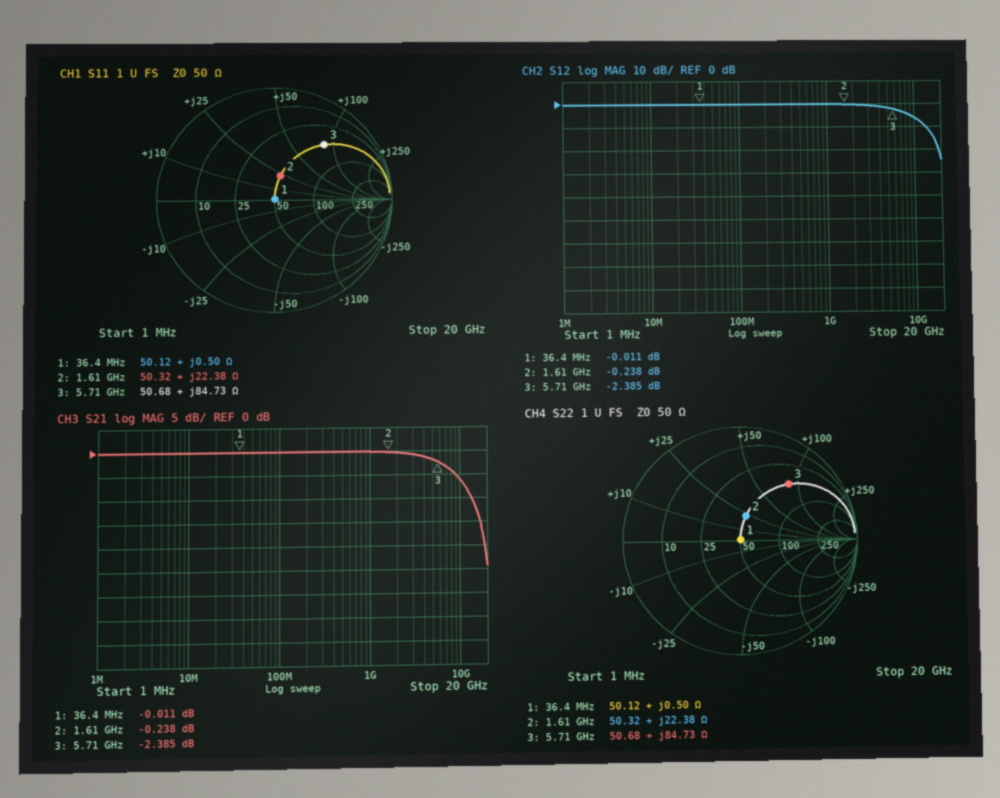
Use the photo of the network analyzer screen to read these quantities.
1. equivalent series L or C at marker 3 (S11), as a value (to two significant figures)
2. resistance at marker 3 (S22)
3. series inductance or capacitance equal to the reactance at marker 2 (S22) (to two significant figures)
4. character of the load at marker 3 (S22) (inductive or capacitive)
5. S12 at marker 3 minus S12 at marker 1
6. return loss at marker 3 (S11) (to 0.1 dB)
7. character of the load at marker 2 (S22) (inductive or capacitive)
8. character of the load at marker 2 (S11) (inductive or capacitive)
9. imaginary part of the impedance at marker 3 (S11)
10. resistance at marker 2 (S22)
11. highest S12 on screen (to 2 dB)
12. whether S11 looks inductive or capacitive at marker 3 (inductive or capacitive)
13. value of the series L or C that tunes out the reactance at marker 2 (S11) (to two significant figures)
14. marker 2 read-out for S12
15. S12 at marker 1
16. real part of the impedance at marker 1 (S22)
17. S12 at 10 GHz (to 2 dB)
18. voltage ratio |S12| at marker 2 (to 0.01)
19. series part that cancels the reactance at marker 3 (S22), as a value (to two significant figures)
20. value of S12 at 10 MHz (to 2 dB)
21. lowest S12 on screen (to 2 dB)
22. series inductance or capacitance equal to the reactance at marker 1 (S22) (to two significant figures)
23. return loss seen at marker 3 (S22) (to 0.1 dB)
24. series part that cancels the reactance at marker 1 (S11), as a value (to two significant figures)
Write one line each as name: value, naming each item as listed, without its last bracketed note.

equivalent series L or C at marker 3 (S11), as a value: 2.4 nH
resistance at marker 3: 50.68 Ω
series inductance or capacitance equal to the reactance at marker 2 (S22): 2.2 nH
character of the load at marker 3 (S22): inductive
S12 at marker 3 minus S12 at marker 1: -2.374 dB
return loss at marker 3 (S11): 3.8 dB
character of the load at marker 2 (S22): inductive
character of the load at marker 2 (S11): inductive
imaginary part of the impedance at marker 3: +84.73 Ω
resistance at marker 2: 50.32 Ω
highest S12 on screen: 0 dB
whether S11 looks inductive or capacitive at marker 3: inductive
value of the series L or C that tunes out the reactance at marker 2 (S11): 4.4 pF
marker 2 read-out for S12: -0.238 dB
S12 at marker 1: -0.011 dB
real part of the impedance at marker 1: 50.12 Ω
S12 at 10 GHz: -6 dB
voltage ratio |S12| at marker 2: 0.97
series part that cancels the reactance at marker 3 (S22), as a value: 330 fF
value of S12 at 10 MHz: 0 dB
lowest S12 on screen: -24 dB
series inductance or capacitance equal to the reactance at marker 1 (S22): 2.2 nH
return loss seen at marker 3 (S22): 3.8 dB
series part that cancels the reactance at marker 1 (S11), as a value: 8.7 nF
